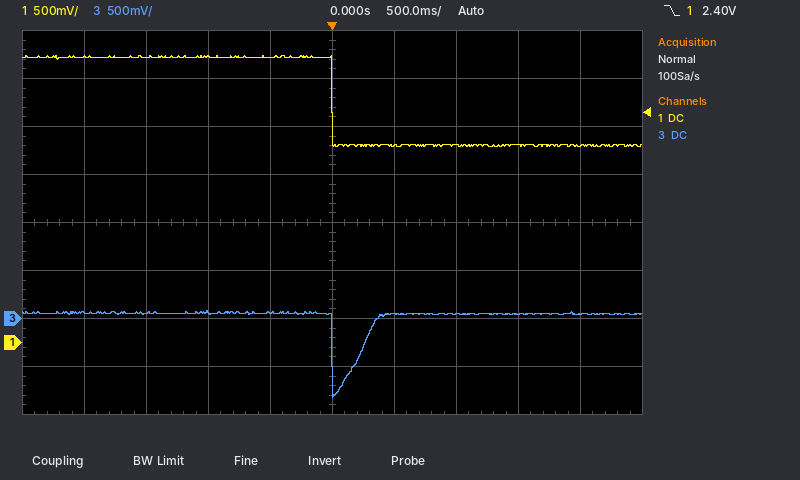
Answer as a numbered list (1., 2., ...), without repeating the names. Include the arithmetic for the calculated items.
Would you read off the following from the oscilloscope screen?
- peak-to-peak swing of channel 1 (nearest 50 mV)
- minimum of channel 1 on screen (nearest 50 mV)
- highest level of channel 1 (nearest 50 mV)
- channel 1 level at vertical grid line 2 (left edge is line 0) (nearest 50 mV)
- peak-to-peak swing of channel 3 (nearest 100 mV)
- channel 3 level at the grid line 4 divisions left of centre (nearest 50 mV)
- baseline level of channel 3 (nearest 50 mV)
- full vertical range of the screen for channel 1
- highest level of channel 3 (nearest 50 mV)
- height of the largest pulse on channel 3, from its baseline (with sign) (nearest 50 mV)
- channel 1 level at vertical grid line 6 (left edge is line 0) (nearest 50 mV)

1. 3.00 V − (2.05 V) = 950 mV
2. 2.05 V
3. 3.00 V
4. 2.95 V
5. 900 mV
6. 50 mV
7. 50 mV
8. 4 V
9. 100 mV
10. -900 mV
11. 2.05 V
